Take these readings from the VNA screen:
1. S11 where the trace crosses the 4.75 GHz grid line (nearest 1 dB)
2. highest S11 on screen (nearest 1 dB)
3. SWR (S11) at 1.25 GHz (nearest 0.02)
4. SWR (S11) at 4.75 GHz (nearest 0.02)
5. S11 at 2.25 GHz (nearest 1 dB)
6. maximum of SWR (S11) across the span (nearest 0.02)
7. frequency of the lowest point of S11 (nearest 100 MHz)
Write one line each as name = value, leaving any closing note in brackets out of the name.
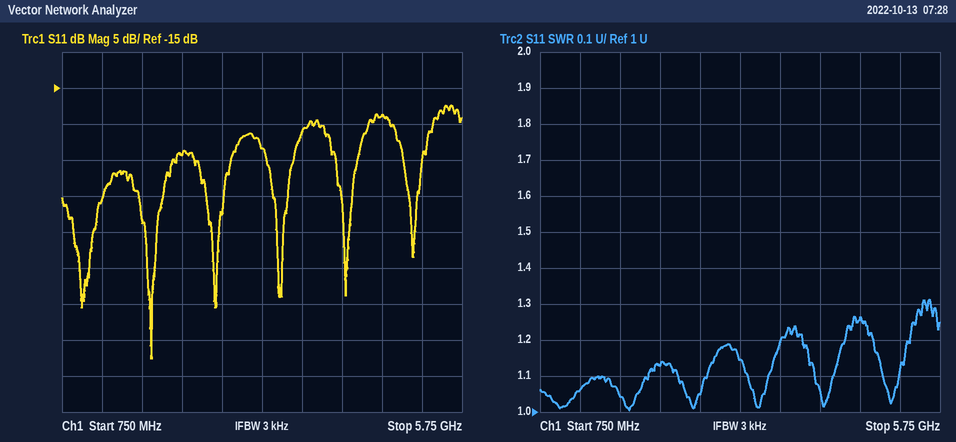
S11 where the trace crosses the 4.75 GHz grid line = -19 dB
highest S11 on screen = -17 dB
SWR (S11) at 1.25 GHz = 1.06
SWR (S11) at 4.75 GHz = 1.26
S11 at 2.25 GHz = -24 dB
maximum of SWR (S11) across the span = 1.32
frequency of the lowest point of S11 = 1.9 GHz
